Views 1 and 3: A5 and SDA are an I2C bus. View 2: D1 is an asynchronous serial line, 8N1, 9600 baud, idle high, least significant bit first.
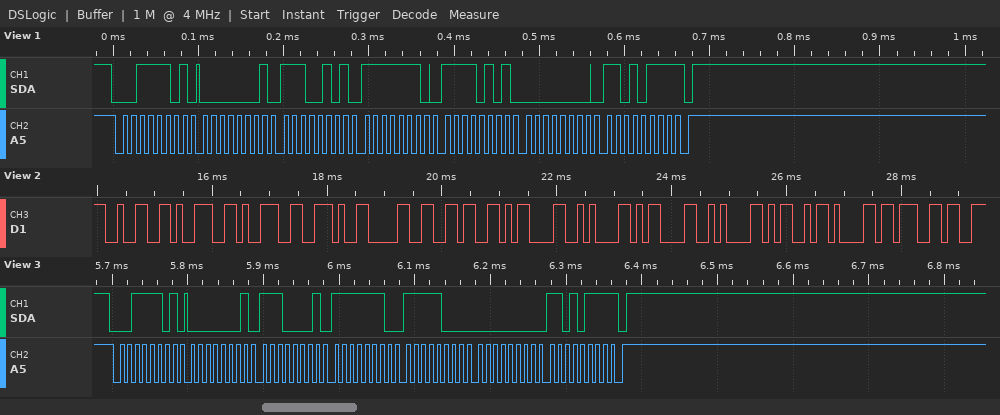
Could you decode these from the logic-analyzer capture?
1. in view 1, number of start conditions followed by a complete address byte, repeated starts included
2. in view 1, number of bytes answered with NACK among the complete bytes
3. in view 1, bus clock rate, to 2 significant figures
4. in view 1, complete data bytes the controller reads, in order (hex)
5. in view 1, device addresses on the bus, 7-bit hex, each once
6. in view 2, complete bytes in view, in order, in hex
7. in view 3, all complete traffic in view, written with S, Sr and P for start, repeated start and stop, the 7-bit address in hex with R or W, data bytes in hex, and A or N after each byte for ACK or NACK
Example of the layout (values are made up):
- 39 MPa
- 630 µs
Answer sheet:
- 1
- 1
- 100 kHz
- 01 E5 FE F5 00 D7
- 0x1E
- 32 39 39 2E 30 36 0D 0A 0D 0A 4D 61 67
- S 1ER A 01 A E1 A FE A F8 A 00 A D7 N P
